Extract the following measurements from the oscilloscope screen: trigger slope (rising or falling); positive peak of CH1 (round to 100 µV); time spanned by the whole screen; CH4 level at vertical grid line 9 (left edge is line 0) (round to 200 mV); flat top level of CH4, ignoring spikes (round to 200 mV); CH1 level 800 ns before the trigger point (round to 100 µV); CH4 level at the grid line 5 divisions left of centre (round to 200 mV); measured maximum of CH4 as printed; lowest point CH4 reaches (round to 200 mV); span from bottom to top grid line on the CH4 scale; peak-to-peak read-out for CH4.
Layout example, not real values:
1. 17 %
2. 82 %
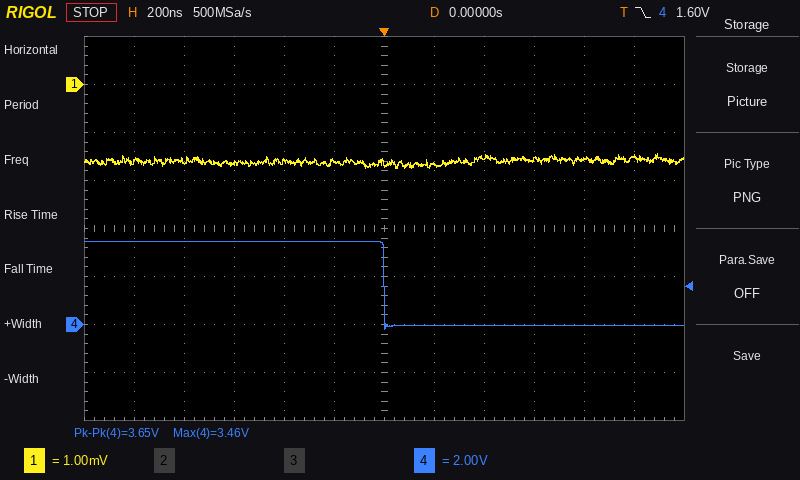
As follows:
1. falling
2. -1.4 mV
3. 2.4 µs
4. 0.0 V
5. 3.4 V
6. -1.6 mV
7. 3.4 V
8. 3.46 V
9. -200 mV
10. 16 V
11. 3.65 V
